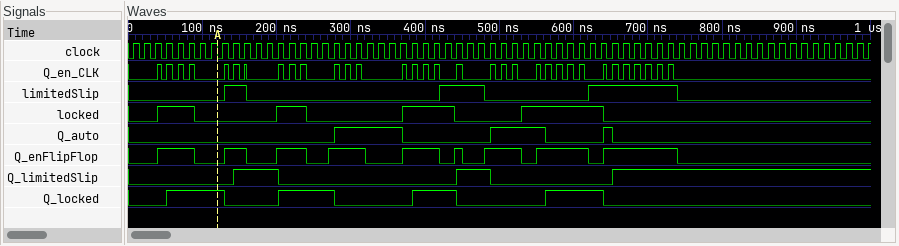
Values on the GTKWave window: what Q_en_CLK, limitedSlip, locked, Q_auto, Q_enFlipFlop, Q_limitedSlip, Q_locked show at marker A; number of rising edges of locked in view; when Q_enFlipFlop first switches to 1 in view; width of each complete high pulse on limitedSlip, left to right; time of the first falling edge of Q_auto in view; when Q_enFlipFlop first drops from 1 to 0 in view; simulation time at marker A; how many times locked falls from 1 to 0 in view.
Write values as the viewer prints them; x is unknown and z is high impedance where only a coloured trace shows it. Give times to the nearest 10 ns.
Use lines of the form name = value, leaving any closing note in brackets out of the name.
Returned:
what Q_en_CLK, limitedSlip, locked, Q_auto, Q_enFlipFlop, Q_limitedSlip, Q_locked show at marker A = Q_en_CLK=0, limitedSlip=0, locked=0, Q_auto=0, Q_enFlipFlop=0, Q_limitedSlip=0, Q_locked=1
number of rising edges of locked in view = 4
when Q_enFlipFlop first switches to 1 in view = 40 ns
width of each complete high pulse on limitedSlip, left to right = 30 ns, 60 ns, 120 ns
time of the first falling edge of Q_auto in view = 370 ns
when Q_enFlipFlop first drops from 1 to 0 in view = 90 ns
simulation time at marker A = 120 ns
how many times locked falls from 1 to 0 in view = 4
